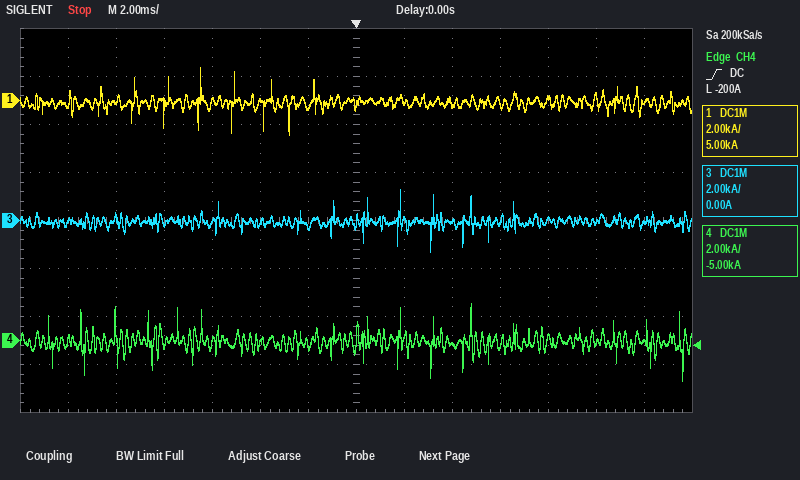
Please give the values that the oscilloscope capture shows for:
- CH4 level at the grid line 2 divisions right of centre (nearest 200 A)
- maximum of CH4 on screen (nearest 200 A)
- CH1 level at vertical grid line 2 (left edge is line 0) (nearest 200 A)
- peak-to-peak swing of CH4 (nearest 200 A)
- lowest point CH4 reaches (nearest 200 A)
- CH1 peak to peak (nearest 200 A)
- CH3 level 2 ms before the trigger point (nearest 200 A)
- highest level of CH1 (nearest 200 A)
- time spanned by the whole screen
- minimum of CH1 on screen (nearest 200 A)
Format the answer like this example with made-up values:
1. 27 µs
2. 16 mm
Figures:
1. -200 A
2. 1.6 kA
3. 0.0 kA
4. 3.2 kA
5. -1.6 kA
6. 2.8 kA
7. -200 A
8. 1.4 kA
9. 28 ms
10. -1.4 kA
